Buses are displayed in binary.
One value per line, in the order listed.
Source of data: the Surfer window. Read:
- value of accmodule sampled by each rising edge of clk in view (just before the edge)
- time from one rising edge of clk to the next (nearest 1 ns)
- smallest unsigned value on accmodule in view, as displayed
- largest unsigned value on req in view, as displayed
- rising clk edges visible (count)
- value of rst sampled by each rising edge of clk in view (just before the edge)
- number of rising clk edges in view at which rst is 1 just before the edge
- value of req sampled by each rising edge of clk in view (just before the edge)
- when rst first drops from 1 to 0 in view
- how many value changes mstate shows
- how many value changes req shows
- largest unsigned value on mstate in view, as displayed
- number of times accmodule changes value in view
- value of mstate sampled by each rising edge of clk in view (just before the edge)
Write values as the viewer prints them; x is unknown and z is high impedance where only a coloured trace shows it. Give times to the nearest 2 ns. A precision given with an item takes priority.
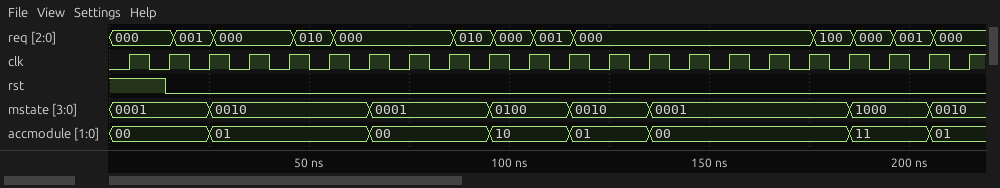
00, 00, 00, 01, 01, 01, 01, 00, 00, 00, 10, 10, 01, 01, 00, 00, 00, 00, 00, 11, 11, 01
10 ns
00
100
22
1 0 0 0 0 0 0 0 0 0 0 0 0 0 0 0 0 0 0 0 0 0
1
000, 000, 001, 000, 000, 010, 000, 000, 000, 010, 000, 001, 000, 000, 000, 000, 000, 000, 100, 000, 001, 000
14 ns
7
12
1000
7
0001, 0001, 0001, 0010, 0010, 0010, 0010, 0001, 0001, 0001, 0100, 0100, 0010, 0010, 0001, 0001, 0001, 0001, 0001, 1000, 1000, 0010
